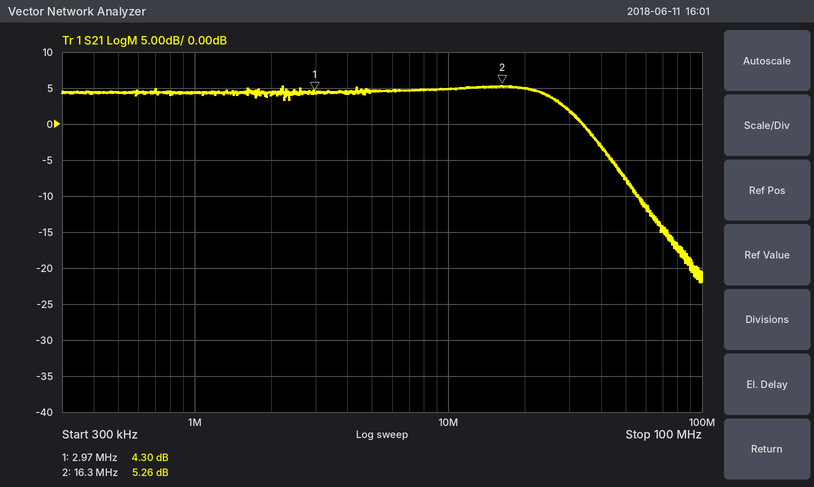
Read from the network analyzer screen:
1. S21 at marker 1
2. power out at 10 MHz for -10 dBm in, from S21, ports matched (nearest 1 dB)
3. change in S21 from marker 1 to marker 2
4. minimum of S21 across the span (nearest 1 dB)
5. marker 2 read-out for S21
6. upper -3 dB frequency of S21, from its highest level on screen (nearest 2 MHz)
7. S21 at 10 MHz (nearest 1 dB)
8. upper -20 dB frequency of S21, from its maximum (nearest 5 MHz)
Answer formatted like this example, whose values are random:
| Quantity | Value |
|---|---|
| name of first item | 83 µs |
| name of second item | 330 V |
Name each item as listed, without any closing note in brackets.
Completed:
| Quantity | Value |
|---|---|
| S21 at marker 1 | 4.30 dB |
| power out at 10 MHz for -10 dBm in, from S21, ports matched | -5 dBm |
| change in S21 from marker 1 to marker 2 | 0.96 dB |
| minimum of S21 across the span | -22 dB |
| marker 2 read-out for S21 | 5.26 dB |
| upper -3 dB frequency of S21, from its highest level on screen | 28 MHz |
| S21 at 10 MHz | 5 dB |
| upper -20 dB frequency of S21, from its maximum | 70 MHz |
